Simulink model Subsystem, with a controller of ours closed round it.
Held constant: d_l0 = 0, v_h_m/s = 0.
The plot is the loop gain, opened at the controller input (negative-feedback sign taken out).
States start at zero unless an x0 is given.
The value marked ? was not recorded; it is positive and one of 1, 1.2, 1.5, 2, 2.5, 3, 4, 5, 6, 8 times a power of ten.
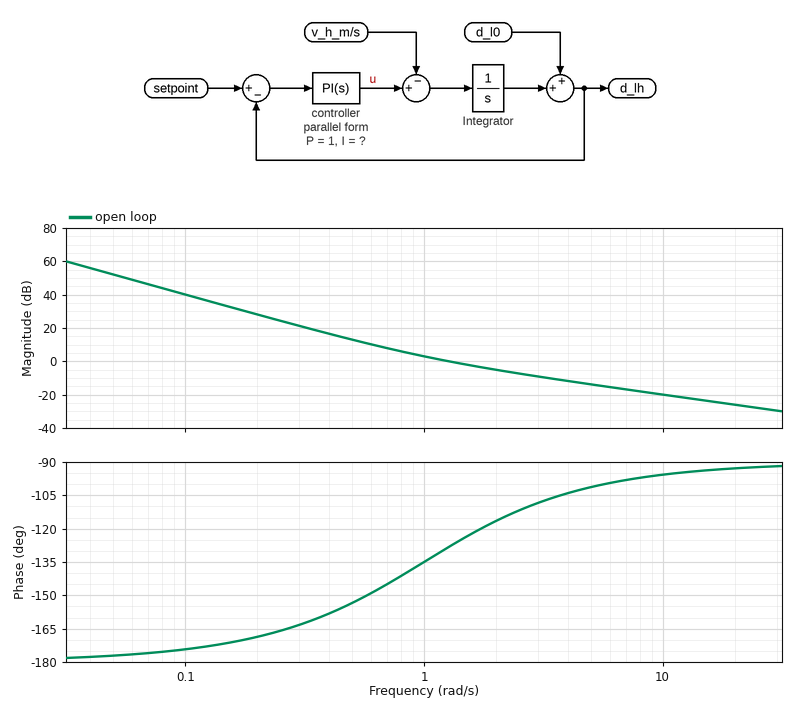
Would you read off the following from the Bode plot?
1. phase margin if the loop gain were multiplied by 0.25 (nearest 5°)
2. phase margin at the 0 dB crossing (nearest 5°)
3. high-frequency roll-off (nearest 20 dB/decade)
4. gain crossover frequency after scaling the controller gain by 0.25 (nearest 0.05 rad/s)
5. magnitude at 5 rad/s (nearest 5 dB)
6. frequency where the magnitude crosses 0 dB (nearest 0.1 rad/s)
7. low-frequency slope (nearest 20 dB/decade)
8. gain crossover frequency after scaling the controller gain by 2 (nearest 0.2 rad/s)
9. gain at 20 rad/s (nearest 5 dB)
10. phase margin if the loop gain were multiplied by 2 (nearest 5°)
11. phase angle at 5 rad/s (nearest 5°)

30°
50°
-20 dB/decade
0.55 rad/s
-15 dB
1.3 rad/s
-40 dB/decade
2.2 rad/s
-25 dB
65°
-100°
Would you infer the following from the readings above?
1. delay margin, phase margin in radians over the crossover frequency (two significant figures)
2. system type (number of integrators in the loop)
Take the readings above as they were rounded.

0.67 s
2
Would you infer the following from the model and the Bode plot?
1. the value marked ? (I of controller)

1
